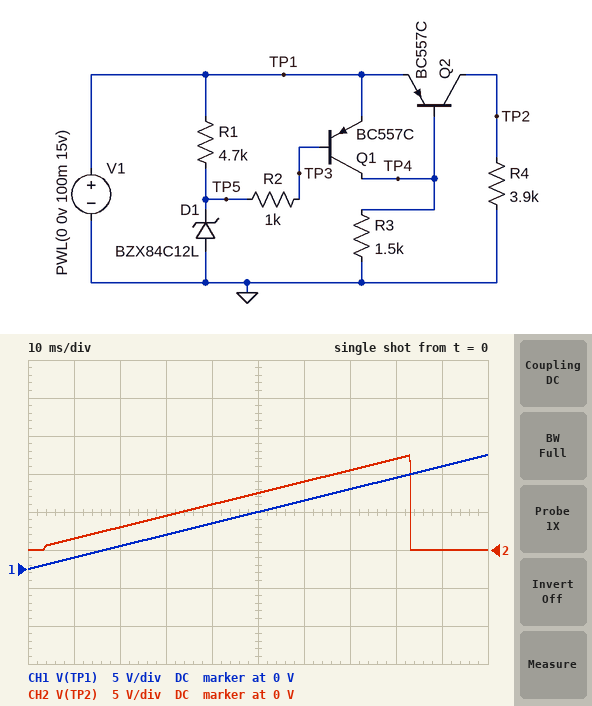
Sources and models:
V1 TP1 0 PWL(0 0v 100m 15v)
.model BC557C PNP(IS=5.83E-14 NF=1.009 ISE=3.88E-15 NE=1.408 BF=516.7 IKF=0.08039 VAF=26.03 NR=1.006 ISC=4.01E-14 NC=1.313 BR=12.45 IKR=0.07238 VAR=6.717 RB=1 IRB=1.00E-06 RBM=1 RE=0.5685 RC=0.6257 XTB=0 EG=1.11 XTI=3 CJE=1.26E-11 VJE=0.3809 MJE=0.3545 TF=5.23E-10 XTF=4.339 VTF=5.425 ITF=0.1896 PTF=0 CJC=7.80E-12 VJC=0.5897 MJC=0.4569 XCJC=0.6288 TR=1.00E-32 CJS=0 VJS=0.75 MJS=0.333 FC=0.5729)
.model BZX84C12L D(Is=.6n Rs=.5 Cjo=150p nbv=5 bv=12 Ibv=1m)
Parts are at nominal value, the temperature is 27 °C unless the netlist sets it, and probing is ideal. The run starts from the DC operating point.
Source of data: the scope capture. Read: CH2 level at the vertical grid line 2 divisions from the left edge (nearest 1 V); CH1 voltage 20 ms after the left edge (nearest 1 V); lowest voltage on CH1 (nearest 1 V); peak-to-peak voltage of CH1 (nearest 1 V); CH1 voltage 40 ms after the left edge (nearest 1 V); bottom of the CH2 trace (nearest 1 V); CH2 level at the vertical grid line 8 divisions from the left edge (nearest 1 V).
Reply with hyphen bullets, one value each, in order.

- 3 V
- 3 V
- 0 V
- 15 V
- 6 V
- 0 V
- 12 V
